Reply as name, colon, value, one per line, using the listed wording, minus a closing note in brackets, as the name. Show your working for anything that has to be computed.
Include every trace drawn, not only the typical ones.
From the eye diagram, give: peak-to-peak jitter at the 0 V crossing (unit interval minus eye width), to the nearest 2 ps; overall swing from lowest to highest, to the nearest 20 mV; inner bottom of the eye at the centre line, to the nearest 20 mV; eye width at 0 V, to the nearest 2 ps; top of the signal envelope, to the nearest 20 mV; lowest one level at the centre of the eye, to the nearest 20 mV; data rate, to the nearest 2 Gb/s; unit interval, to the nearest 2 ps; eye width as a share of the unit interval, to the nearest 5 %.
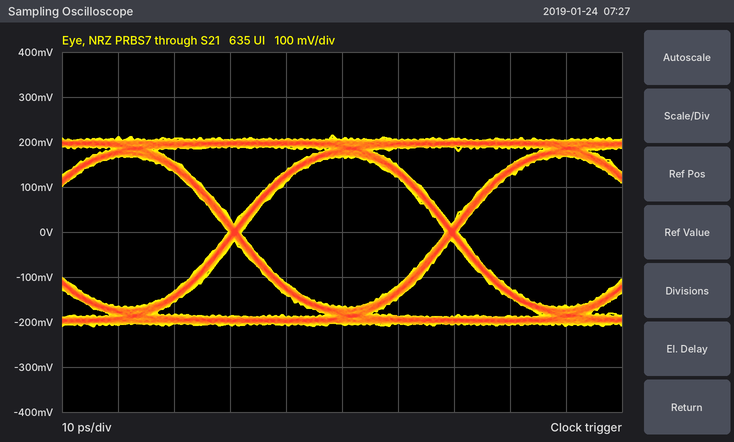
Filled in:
peak-to-peak jitter at the 0 V crossing (unit interval minus eye width), to the nearest 2 ps: 2 ps
overall swing from lowest to highest, to the nearest 20 mV: 420 mV
inner bottom of the eye at the centre line, to the nearest 20 mV: -160 mV
eye width at 0 V, to the nearest 2 ps: 36 ps
top of the signal envelope, to the nearest 20 mV: 220 mV
lowest one level at the centre of the eye, to the nearest 20 mV: 160 mV
data rate, to the nearest 2 Gb/s: 26 Gb/s
unit interval, to the nearest 2 ps: 38 ps
eye width as a share of the unit interval, to the nearest 5 %: 36 ps / 38 ps ≈ 95 %
